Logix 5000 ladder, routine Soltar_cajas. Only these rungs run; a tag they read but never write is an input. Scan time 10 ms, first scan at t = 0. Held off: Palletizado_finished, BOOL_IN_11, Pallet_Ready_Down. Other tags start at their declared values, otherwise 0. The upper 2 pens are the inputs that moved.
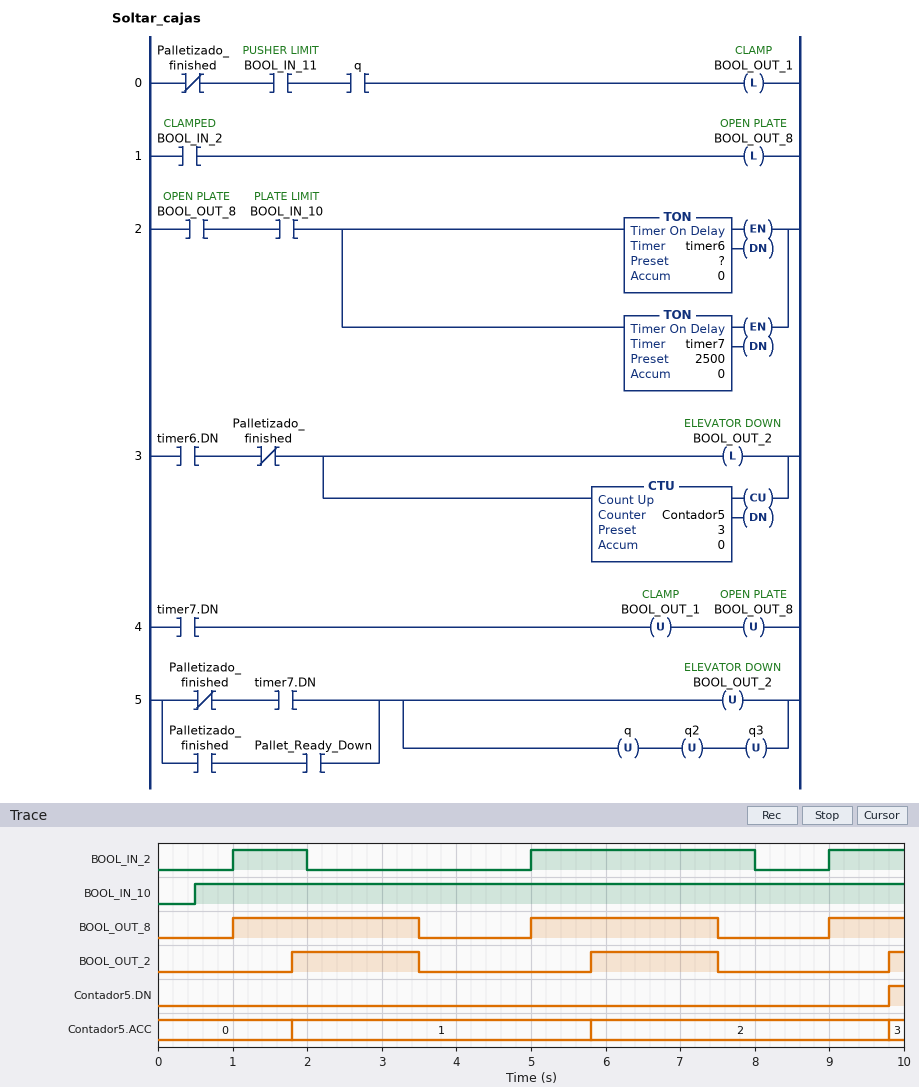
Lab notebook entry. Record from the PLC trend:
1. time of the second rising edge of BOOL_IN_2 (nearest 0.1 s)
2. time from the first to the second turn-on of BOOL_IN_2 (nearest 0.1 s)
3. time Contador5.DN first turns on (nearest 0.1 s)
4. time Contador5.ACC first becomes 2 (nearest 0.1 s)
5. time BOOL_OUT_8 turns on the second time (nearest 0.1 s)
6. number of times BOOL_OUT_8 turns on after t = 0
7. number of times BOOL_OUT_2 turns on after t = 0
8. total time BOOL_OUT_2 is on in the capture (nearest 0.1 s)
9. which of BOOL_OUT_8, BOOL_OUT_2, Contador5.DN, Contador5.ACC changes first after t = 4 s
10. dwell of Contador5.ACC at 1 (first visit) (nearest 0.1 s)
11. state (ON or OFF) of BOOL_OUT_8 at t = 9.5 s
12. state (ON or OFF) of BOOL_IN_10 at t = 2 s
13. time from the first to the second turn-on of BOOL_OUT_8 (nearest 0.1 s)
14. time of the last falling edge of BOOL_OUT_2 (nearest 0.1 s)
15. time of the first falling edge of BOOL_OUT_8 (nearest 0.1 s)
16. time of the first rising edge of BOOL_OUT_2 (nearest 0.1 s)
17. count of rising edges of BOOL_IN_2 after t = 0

5.0 s
4.0 s
9.8 s
5.8 s
5.0 s
3
3
3.6 s
BOOL_OUT_8
4.0 s
ON
ON
4.0 s
7.5 s
3.5 s
1.8 s
3
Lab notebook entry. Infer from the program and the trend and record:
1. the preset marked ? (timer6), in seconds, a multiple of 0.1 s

0.8 s
